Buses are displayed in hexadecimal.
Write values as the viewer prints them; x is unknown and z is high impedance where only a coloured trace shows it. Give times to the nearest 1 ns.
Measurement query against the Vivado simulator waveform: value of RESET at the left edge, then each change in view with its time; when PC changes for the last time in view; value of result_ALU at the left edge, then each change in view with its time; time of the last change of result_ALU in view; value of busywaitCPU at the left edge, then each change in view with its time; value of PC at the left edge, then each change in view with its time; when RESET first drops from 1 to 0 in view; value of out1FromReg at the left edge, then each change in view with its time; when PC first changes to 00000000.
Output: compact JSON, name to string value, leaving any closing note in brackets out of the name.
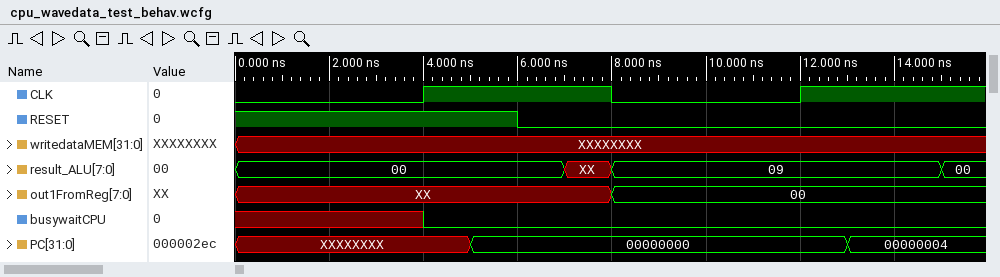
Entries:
{"value of RESET at the left edge, then each change in view with its time": "1, 0 at 6 ns", "when PC changes for the last time in view": "13 ns", "value of result_ALU at the left edge, then each change in view with its time": "00, XX at 7 ns, 09 at 8 ns, 00 at 15 ns", "time of the last change of result_ALU in view": "15 ns", "value of busywaitCPU at the left edge, then each change in view with its time": "x, 0 at 4 ns", "value of PC at the left edge, then each change in view with its time": "XXXXXXXX, 00000000 at 5 ns, 00000004 at 13 ns", "when RESET first drops from 1 to 0 in view": "6 ns", "value of out1FromReg at the left edge, then each change in view with its time": "XX, 00 at 8 ns", "when PC first changes to 00000000": "5 ns"}
